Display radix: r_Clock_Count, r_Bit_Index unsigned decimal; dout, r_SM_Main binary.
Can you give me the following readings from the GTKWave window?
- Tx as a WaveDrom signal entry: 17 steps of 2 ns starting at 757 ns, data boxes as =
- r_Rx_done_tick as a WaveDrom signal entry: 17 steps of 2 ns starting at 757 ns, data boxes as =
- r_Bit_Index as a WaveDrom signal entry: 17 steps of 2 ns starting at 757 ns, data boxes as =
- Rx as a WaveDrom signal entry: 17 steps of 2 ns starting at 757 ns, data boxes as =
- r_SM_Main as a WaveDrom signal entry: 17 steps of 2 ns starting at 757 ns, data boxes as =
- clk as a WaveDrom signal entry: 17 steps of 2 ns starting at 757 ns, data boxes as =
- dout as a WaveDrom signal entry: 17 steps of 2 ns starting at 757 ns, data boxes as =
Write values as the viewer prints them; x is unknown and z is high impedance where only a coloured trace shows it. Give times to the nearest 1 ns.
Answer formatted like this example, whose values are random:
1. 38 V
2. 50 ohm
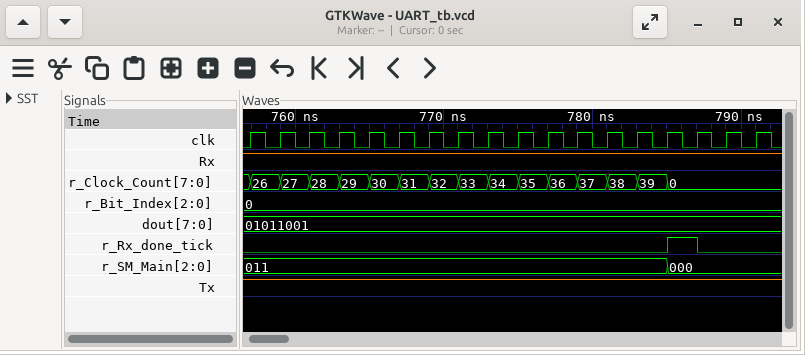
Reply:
1. {name: 'Tx', wave: '1................'}
2. {name: 'r_Rx_done_tick', wave: '0.............10.'}
3. {name: 'r_Bit_Index', wave: '=................', data: '0'}
4. {name: 'Rx', wave: '1................'}
5. {name: 'r_SM_Main', wave: '=.............=..', data: '011 000'}
6. {name: 'clk', wave: 'p................'}
7. {name: 'dout', wave: '=................', data: '01011001'}
